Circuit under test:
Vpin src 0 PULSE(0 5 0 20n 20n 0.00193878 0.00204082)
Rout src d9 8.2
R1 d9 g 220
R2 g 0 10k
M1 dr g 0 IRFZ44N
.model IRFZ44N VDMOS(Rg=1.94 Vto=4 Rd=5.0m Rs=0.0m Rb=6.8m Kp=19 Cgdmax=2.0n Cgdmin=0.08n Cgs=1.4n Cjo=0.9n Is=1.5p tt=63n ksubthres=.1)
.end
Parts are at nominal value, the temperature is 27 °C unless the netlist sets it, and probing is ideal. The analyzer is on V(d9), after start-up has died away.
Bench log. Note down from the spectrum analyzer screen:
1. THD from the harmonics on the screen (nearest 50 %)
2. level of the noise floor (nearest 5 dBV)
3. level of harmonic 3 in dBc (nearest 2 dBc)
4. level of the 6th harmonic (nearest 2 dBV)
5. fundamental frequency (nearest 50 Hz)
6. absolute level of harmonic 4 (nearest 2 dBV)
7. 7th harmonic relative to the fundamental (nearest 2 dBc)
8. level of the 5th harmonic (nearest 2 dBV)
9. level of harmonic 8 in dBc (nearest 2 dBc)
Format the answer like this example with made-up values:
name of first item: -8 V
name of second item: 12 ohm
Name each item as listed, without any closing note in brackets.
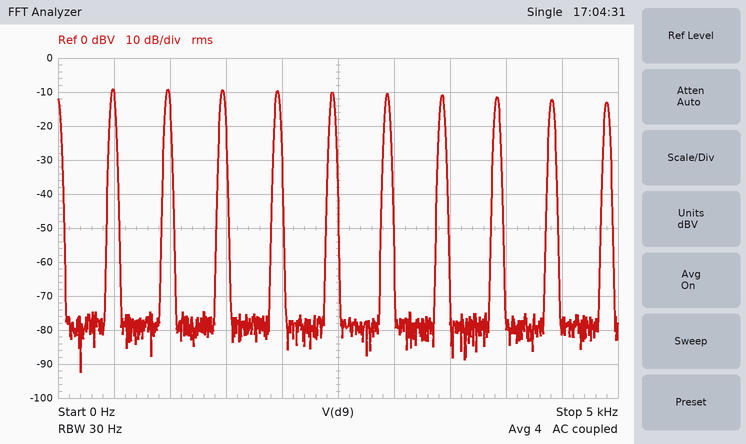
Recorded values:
THD from the harmonics on the screen: 250 %
level of the noise floor: -80 dBV
level of harmonic 3 in dBc: 0 dBc
level of the 6th harmonic: -10 dBV
fundamental frequency: 500 Hz
absolute level of harmonic 4: -10 dBV
7th harmonic relative to the fundamental: -2 dBc
level of the 5th harmonic: -10 dBV
level of harmonic 8 in dBc: -2 dBc
